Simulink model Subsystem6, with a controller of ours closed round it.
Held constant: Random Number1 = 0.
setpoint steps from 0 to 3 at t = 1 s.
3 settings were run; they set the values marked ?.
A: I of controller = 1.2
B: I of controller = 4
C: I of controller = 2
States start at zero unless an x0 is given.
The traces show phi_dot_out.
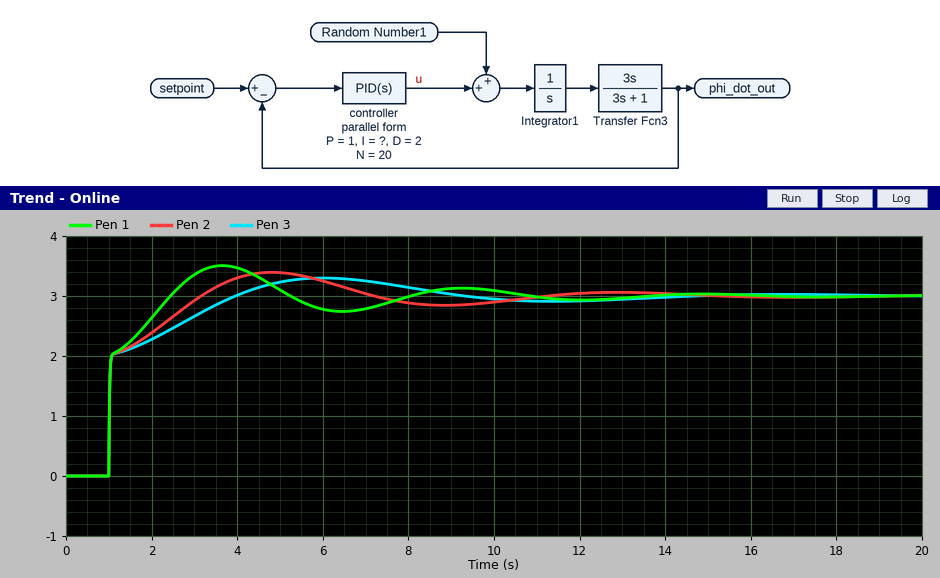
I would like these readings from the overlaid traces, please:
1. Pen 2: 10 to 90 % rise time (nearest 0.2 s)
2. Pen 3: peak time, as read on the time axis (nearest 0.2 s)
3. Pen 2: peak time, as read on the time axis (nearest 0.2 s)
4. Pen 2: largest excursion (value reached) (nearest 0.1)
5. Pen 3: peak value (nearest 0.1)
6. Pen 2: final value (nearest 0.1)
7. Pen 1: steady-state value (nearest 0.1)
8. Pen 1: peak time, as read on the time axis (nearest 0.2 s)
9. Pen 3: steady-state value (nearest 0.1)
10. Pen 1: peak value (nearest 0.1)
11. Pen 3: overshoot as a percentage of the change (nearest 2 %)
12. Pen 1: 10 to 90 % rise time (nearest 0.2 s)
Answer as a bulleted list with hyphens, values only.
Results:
- 1.6 s
- 6.0 s
- 4.8 s
- 3.4
- 3.3
- 3.0
- 3.0
- 3.6 s
- 3.0
- 3.5
- 10 %
- 1.0 s
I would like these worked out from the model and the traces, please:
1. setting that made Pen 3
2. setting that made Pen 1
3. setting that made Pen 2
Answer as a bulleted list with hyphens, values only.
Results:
- A
- B
- C
